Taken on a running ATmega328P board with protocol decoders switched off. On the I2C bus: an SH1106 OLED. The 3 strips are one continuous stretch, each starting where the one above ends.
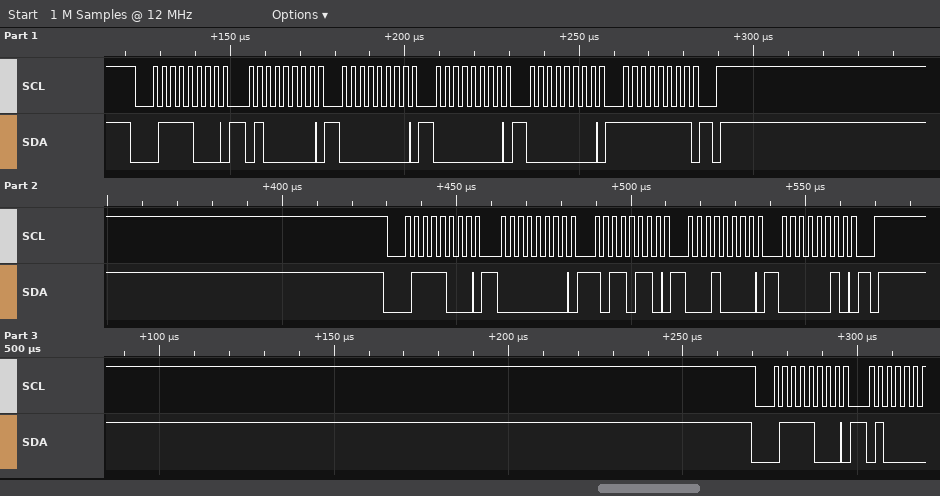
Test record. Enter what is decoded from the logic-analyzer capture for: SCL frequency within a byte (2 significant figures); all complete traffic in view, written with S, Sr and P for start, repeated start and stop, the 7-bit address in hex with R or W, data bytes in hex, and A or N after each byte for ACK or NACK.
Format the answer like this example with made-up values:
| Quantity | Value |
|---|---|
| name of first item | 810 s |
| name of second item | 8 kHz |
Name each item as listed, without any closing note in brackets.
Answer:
| Quantity | Value |
|---|---|
| SCL frequency within a byte | 400 kHz |
| all complete traffic in view, written with S, Sr and P for start, repeated start and stop, the 7-bit address in hex with R or W, data bytes in hex, and A or N after each byte for ACK or NACK | S 3CW A 40 A 00 A 00 A 00 A FF A P S 3CW A 00 A B6 A 10 A 02 A P S 3CW A |
